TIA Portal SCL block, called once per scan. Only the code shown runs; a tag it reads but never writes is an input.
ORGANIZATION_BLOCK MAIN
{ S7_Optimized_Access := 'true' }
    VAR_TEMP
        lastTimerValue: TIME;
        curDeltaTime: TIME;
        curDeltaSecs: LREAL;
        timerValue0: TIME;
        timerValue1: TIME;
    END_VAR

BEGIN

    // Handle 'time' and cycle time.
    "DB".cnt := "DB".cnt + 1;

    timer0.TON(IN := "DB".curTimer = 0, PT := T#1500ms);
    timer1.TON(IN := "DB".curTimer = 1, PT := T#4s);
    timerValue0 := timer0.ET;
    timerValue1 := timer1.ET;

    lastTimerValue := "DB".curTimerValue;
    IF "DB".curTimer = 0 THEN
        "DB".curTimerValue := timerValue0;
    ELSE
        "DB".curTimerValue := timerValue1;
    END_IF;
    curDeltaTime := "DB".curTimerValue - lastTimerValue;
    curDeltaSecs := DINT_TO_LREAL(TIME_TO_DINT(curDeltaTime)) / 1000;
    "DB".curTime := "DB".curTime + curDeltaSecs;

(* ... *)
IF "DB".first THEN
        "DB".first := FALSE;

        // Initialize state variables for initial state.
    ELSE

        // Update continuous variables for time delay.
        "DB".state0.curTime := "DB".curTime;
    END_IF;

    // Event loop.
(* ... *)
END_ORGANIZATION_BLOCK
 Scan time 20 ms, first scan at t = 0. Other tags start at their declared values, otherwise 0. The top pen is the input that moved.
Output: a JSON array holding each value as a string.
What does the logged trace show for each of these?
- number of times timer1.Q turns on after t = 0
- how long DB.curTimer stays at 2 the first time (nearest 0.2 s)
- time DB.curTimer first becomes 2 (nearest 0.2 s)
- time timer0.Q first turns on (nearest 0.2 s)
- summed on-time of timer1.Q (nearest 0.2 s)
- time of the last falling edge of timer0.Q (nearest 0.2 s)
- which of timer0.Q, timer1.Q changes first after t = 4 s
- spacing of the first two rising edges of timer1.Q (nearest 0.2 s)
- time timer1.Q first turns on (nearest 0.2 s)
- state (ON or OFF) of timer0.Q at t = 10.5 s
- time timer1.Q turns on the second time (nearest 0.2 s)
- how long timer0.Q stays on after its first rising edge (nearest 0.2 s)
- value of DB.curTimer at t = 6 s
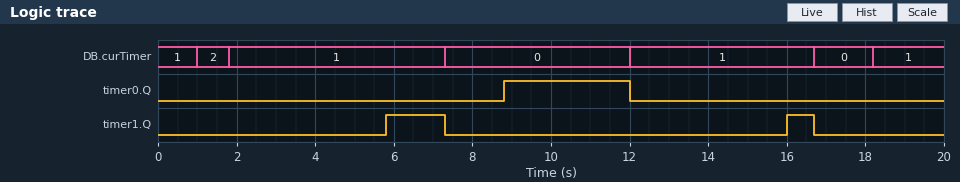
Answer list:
["2", "0.8 s", "1.0 s", "8.8 s", "2.2 s", "12.0 s", "timer1.Q", "10.2 s", "5.8 s", "ON", "16.0 s", "3.2 s", "1"]
